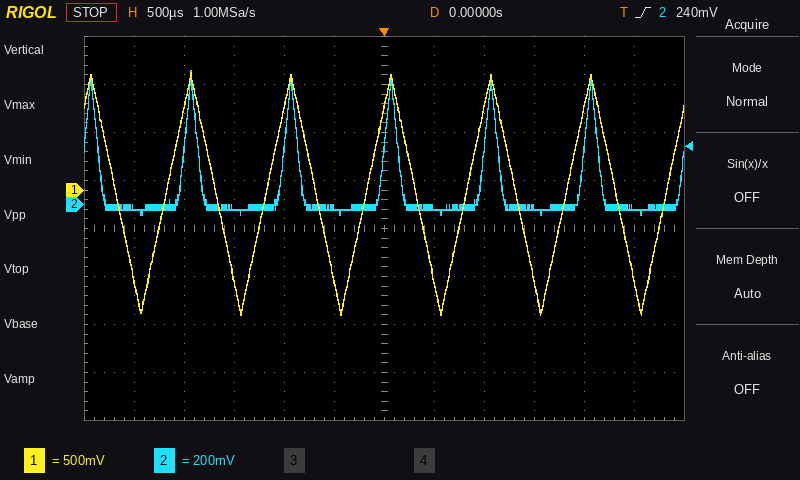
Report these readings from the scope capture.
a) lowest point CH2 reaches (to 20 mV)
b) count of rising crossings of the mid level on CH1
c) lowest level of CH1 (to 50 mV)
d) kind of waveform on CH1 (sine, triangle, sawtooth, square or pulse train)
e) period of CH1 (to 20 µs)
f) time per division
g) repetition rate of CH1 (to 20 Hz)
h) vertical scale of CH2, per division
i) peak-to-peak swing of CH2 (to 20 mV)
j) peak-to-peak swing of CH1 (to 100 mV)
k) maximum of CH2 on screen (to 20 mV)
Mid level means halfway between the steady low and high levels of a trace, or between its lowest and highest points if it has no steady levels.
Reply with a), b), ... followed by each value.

a) -40 mV
b) 6
c) -1.30 V
d) triangle
e) 1.00 ms
f) 500 µs
g) 1.00 kHz
h) 200 mV
i) 600 mV
j) 2.50 V
k) 560 mV
